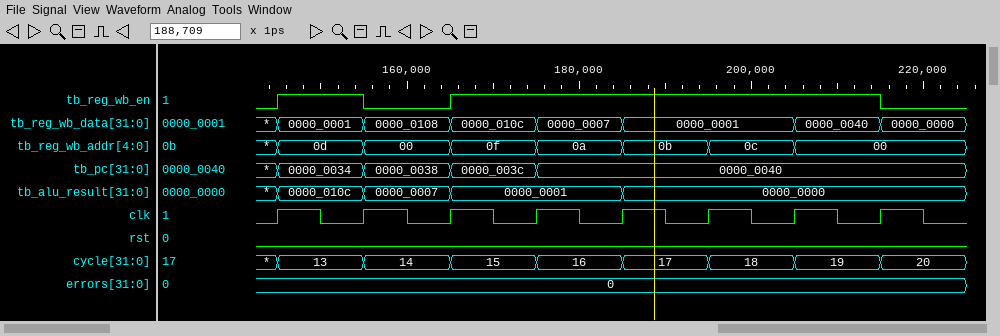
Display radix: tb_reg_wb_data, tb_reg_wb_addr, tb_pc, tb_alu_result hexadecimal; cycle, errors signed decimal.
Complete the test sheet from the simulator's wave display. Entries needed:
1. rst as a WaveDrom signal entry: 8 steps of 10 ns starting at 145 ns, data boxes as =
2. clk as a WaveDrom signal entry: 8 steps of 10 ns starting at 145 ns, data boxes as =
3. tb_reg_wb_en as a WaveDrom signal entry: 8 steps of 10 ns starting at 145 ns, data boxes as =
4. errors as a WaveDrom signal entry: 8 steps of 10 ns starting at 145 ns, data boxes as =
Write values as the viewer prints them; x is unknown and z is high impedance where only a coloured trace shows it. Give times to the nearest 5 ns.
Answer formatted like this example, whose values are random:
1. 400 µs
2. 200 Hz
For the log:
1. {name: 'rst', wave: '0.......'}
2. {name: 'clk', wave: 'p.......'}
3. {name: 'tb_reg_wb_en', wave: '101....0'}
4. {name: 'errors', wave: '=.......', data: '0'}
